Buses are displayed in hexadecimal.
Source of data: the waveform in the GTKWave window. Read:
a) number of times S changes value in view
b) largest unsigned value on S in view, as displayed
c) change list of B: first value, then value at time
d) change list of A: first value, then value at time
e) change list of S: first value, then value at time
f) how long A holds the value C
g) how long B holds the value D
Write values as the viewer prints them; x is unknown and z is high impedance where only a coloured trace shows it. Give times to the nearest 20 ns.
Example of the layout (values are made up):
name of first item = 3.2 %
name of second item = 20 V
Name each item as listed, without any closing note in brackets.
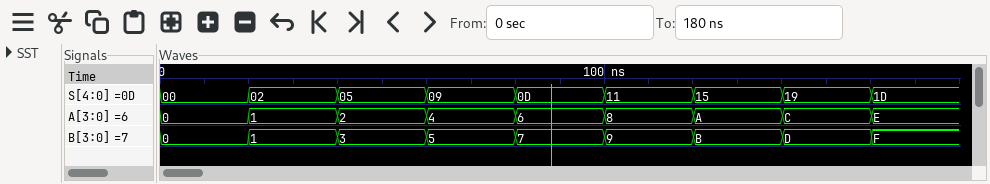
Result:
number of times S changes value in view = 8
largest unsigned value on S in view, as displayed = 1D
change list of B: first value, then value at time = 0, 1 at 20 ns, 3 at 40 ns, 5 at 60 ns, 7 at 80 ns, 9 at 100 ns, B at 120 ns, D at 140 ns, F at 160 ns
change list of A: first value, then value at time = 0, 1 at 20 ns, 2 at 40 ns, 4 at 60 ns, 6 at 80 ns, 8 at 100 ns, A at 120 ns, C at 140 ns, E at 160 ns
change list of S: first value, then value at time = 00, 02 at 20 ns, 05 at 40 ns, 09 at 60 ns, 0D at 80 ns, 11 at 100 ns, 15 at 120 ns, 19 at 140 ns, 1D at 160 ns
how long A holds the value C = 20 ns
how long B holds the value D = 20 ns
